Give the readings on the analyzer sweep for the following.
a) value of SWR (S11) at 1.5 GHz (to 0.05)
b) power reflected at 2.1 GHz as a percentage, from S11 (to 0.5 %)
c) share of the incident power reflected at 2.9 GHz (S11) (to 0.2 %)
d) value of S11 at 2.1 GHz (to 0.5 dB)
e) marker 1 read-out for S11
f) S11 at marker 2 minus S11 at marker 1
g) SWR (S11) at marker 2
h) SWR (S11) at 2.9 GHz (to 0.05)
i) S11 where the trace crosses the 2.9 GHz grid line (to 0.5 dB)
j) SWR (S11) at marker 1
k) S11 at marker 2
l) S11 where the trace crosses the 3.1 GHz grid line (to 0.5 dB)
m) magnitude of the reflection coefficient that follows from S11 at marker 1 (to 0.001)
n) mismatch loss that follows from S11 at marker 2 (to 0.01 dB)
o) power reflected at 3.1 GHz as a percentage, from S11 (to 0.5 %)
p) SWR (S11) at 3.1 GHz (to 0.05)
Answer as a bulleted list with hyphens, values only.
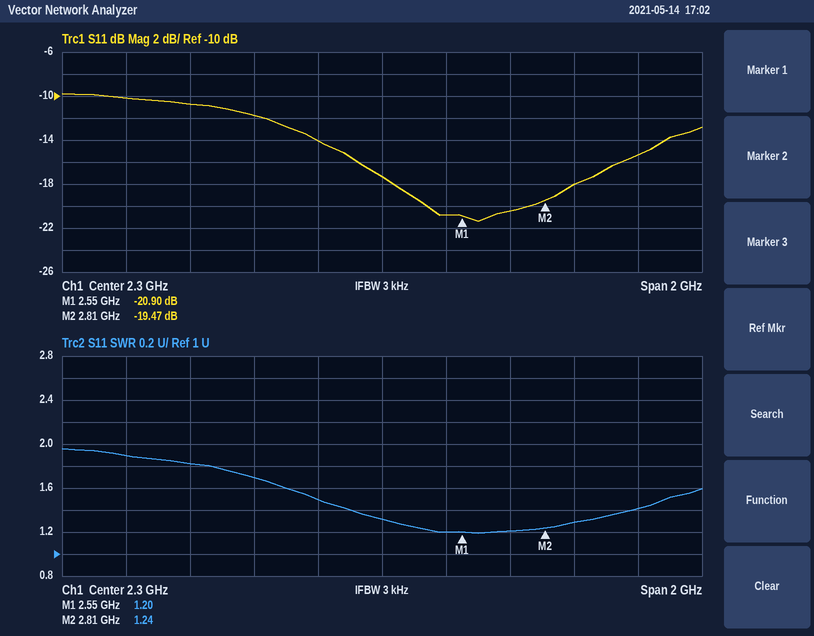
- 1.90
- 4.0 %
- 1.6 %
- -14.0 dB
- -20.90 dB
- 1.43 dB
- 1.24
- 1.30
- -18.0 dB
- 1.20
- -19.47 dB
- -15.5 dB
- 0.090
- 0.05 dB
- 3.0 %
- 1.40
